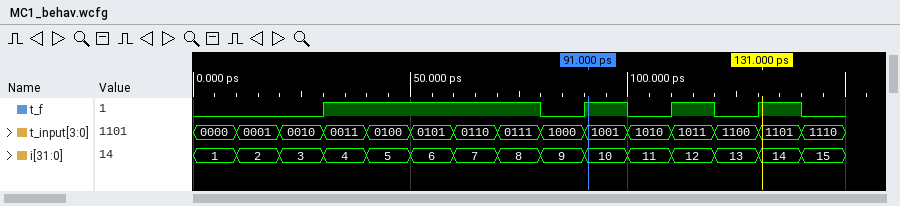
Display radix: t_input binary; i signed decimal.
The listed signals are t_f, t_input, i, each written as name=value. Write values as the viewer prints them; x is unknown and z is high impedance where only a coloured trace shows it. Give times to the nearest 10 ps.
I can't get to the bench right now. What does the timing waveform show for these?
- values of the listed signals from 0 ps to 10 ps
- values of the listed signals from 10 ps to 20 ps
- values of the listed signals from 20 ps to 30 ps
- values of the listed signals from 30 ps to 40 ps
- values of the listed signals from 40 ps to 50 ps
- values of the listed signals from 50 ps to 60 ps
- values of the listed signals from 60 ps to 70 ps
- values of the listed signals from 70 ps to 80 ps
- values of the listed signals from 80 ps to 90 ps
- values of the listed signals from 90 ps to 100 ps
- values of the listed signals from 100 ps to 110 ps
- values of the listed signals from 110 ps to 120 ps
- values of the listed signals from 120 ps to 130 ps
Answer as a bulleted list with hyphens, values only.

- t_f=0, t_input=0000, i=1
- t_f=0, t_input=0001, i=2
- t_f=0, t_input=0010, i=3
- t_f=1, t_input=0011, i=4
- t_f=1, t_input=0100, i=5
- t_f=1, t_input=0101, i=6
- t_f=1, t_input=0110, i=7
- t_f=1, t_input=0111, i=8
- t_f=0, t_input=1000, i=9
- t_f=1, t_input=1001, i=10
- t_f=0, t_input=1010, i=11
- t_f=1, t_input=1011, i=12
- t_f=0, t_input=1100, i=13
